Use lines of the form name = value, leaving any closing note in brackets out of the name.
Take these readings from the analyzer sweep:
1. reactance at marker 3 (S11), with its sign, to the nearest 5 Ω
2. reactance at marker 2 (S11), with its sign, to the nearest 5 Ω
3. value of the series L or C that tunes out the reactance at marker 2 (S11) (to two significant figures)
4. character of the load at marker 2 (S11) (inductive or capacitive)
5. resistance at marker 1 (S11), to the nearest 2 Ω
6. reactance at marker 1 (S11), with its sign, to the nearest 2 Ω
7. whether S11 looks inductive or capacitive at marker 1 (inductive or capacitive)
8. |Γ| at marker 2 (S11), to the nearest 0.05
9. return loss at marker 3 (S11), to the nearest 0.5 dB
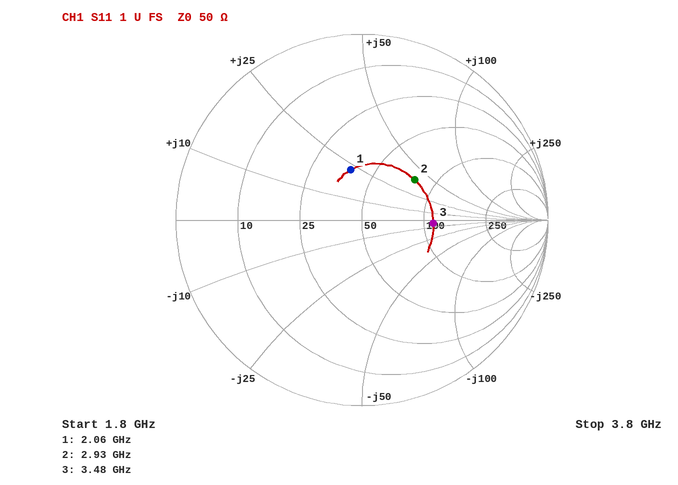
reactance at marker 3 (S11), with its sign, to the nearest 5 Ω = -5 Ω
reactance at marker 2 (S11), with its sign, to the nearest 5 Ω = +40 Ω
value of the series L or C that tunes out the reactance at marker 2 (S11) = 1.4 pF
character of the load at marker 2 (S11) = inductive
resistance at marker 1 (S11), to the nearest 2 Ω = 38 Ω
reactance at marker 1 (S11), with its sign, to the nearest 2 Ω = +22 Ω
whether S11 looks inductive or capacitive at marker 1 = inductive
|Γ| at marker 2 (S11), to the nearest 0.05 = 0.35
return loss at marker 3 (S11), to the nearest 0.5 dB = 8.5 dB
